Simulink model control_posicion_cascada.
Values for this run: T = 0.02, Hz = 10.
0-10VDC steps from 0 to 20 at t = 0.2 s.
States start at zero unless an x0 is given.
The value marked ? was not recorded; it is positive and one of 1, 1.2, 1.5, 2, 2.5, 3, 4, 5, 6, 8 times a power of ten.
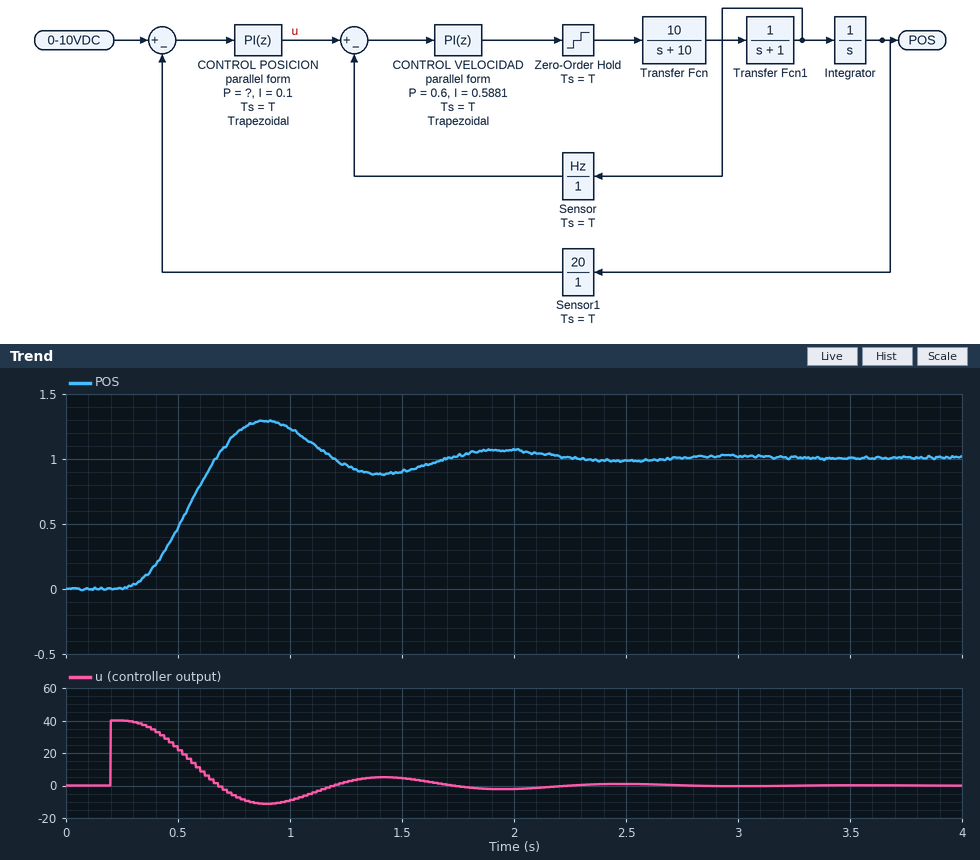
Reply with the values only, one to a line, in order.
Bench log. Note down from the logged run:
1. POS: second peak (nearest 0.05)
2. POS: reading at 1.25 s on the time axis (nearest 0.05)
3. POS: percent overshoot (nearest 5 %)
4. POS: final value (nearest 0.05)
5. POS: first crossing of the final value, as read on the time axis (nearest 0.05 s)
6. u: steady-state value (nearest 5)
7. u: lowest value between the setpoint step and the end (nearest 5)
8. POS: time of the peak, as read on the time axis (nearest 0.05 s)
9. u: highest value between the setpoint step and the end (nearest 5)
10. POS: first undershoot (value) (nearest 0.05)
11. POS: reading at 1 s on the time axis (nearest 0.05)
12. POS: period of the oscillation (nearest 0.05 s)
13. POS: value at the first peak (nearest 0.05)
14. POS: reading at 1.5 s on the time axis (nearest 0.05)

1.05
0.95
30 %
1.00
0.65 s
0
-10
0.90 s
40
0.90
1.25
1.05 s
1.30
0.90
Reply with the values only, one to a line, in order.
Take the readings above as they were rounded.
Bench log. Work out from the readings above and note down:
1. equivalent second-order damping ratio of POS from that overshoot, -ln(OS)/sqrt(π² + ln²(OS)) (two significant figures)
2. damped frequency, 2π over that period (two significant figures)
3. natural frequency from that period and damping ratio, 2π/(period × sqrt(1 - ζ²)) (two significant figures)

0.36
6.0 rad/s
6.4 rad/s
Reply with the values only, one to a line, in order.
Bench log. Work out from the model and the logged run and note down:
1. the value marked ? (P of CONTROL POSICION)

2
